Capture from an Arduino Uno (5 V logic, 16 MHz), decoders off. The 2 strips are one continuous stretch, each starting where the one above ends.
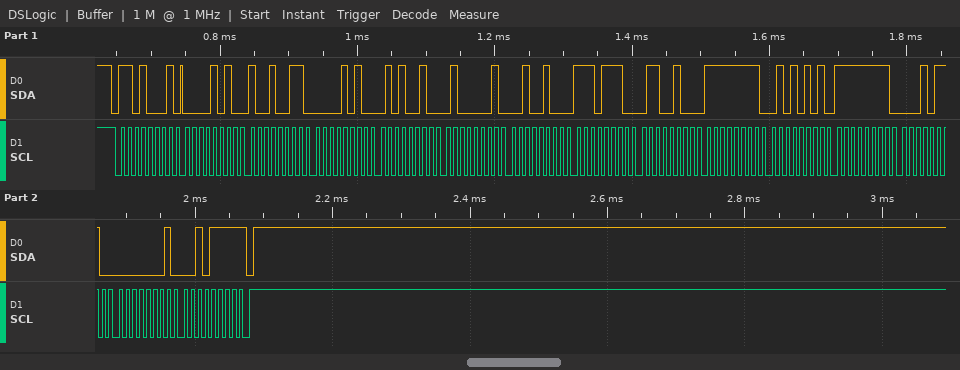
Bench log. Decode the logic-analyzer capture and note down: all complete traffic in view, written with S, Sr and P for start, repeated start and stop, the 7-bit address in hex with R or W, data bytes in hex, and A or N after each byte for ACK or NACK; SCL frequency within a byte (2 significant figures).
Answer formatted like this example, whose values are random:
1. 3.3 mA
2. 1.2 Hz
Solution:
1. S 68R A 0A A 93 A 0A A 52 A 41 A 24 A EE A 64 A FF A 55 A FF A 16 A 01 A 2F N P
2. 100 kHz
